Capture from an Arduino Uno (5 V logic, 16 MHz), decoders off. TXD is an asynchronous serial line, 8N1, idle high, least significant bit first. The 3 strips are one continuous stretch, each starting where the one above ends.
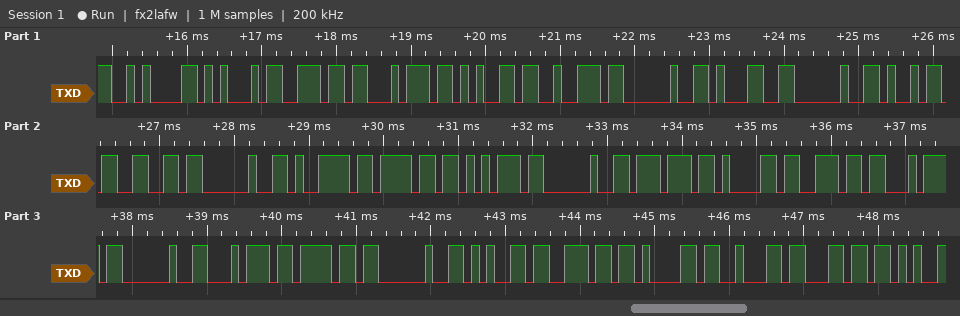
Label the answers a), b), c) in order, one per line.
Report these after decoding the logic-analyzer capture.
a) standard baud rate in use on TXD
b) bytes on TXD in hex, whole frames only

a) 9600 baud
b) 0A 45 6E 74 65 72 20 31 20 69 66 20 79 6F 75 20 77 61 6E 74 20 74 6F 20 65 6E 61 62 6C
